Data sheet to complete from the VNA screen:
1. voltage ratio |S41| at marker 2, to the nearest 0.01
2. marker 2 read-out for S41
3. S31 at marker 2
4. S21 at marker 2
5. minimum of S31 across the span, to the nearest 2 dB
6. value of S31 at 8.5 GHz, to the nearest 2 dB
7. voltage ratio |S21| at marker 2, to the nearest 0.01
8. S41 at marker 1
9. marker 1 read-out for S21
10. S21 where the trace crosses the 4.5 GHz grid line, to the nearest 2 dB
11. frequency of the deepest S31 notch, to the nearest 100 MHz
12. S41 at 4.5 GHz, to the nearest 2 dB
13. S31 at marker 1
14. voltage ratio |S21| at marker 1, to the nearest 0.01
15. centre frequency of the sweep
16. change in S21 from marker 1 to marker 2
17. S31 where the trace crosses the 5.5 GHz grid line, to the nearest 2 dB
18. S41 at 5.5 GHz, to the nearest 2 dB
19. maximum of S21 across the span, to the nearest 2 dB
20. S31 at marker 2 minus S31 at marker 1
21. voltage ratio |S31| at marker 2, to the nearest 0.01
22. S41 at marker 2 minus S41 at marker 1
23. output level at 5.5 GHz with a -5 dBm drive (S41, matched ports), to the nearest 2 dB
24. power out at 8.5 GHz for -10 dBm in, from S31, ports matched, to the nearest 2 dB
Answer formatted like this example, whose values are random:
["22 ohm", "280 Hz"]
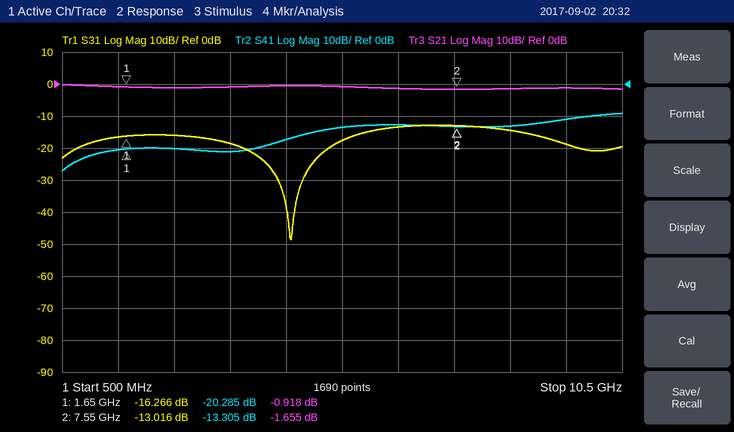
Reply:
["0.22", "-13.305 dB", "-13.016 dB", "-1.655 dB", "-48 dB", "-14 dB", "0.83", "-20.285 dB", "-0.918 dB", "0 dB", "4.6 GHz", "-18 dB", "-16.266 dB", "0.90", "5.5 GHz", "-0.737 dB", "-18 dB", "-14 dB", "0 dB", "3.250 dB", "0.22", "6.980 dB", "-18 dBm", "-24 dBm"]
